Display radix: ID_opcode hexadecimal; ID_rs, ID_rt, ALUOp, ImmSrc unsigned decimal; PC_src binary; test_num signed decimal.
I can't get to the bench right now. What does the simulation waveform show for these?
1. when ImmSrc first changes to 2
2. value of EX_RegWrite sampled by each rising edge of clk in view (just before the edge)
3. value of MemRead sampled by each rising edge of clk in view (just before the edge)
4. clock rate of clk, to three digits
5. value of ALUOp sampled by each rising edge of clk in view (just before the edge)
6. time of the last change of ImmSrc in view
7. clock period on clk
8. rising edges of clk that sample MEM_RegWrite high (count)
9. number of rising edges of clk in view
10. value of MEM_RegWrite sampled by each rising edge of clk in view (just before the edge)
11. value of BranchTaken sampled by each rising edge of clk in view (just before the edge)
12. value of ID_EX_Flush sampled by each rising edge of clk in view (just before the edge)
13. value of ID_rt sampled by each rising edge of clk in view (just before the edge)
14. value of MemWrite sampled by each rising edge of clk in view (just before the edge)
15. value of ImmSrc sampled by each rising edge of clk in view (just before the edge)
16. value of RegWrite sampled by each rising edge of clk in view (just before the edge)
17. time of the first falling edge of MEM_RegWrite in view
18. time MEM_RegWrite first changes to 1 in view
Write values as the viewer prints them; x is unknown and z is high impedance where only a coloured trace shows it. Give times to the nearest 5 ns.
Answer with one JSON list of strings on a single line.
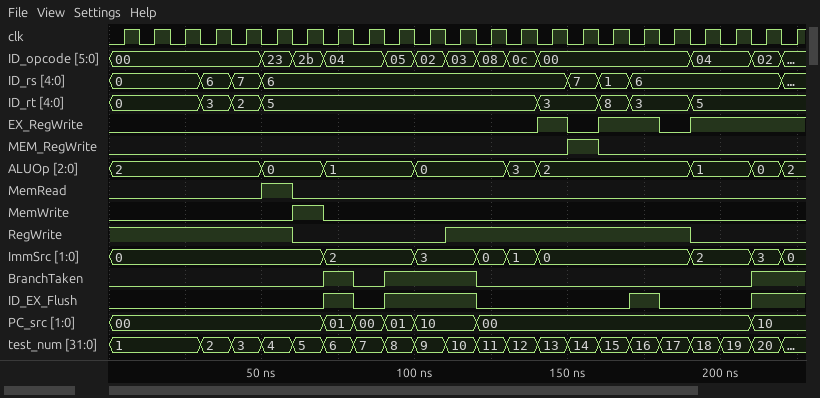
["70 ns", "0 0 0 0 0 0 0 0 0 0 0 0 0 0 1 0 1 1 0 1 1 1 1", "0 0 0 0 0 1 0 0 0 0 0 0 0 0 0 0 0 0 0 0 0 0 0", "100 MHz", "2, 2, 2, 2, 2, 0, 0, 1, 1, 1, 0, 0, 0, 3, 2, 2, 2, 2, 2, 1, 1, 0, 2", "220 ns", "10 ns", "1", "23", "0 0 0 0 0 0 0 0 0 0 0 0 0 0 0 1 0 0 0 0 0 0 0", "0 0 0 0 0 0 0 1 0 1 1 1 0 0 0 0 0 0 0 0 0 1 1", "0 0 0 0 0 0 0 1 0 1 1 1 0 0 0 0 0 1 0 0 0 1 1", "0, 0, 0, 3, 2, 5, 5, 5, 5, 5, 5, 5, 5, 5, 3, 3, 8, 3, 3, 5, 5, 5, 5", "0 0 0 0 0 0 1 0 0 0 0 0 0 0 0 0 0 0 0 0 0 0 0", "0, 0, 0, 0, 0, 0, 0, 2, 2, 2, 3, 3, 0, 1, 0, 0, 0, 0, 0, 2, 2, 3, 0", "1 1 1 1 1 1 0 0 0 0 0 1 1 1 1 1 1 1 1 0 0 0 0", "160 ns", "150 ns"]
